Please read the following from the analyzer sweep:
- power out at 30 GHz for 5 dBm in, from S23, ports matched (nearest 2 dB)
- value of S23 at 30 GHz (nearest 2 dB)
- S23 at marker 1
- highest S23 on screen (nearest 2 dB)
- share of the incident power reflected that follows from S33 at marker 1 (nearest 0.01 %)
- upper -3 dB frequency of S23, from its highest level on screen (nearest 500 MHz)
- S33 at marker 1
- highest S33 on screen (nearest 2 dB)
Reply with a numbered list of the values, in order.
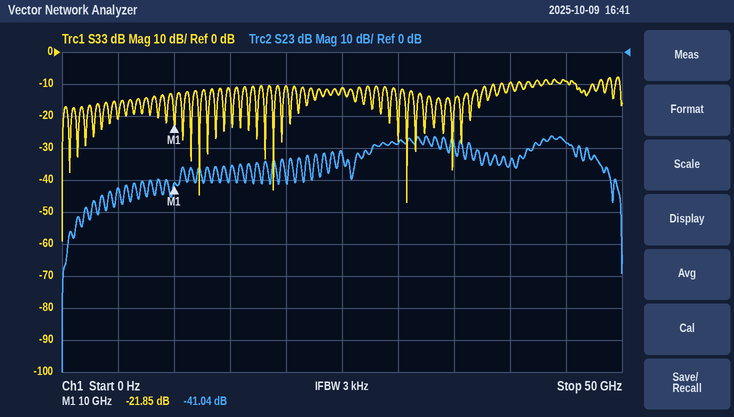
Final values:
1. -24 dBm
2. -28 dB
3. -41.04 dB
4. -26 dB
5. 0.65 %
6. 45.5 GHz
7. -21.85 dB
8. -8 dB
